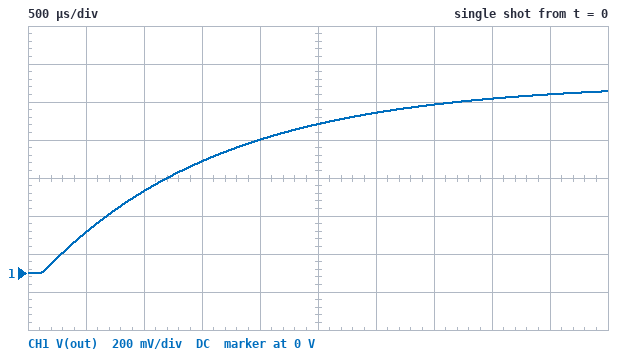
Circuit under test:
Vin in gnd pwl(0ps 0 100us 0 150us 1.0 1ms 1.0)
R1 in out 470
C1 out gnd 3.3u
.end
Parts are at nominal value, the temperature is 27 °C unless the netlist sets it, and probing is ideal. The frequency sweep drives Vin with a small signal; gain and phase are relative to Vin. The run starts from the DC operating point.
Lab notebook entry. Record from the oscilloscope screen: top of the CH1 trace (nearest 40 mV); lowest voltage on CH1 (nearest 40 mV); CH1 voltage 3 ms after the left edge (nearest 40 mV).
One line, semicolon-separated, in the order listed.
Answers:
960 mV; 0 V; 840 mV
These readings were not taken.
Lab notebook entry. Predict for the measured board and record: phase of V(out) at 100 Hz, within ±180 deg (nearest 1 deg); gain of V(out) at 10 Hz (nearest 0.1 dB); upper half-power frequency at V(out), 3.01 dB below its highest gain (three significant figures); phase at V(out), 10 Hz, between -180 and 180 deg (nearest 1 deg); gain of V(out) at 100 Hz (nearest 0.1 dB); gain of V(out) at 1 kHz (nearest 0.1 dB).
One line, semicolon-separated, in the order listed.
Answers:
-44 deg; 0 dB; 103 Hz; -6 deg; -2.9 dB; -19.8 dB
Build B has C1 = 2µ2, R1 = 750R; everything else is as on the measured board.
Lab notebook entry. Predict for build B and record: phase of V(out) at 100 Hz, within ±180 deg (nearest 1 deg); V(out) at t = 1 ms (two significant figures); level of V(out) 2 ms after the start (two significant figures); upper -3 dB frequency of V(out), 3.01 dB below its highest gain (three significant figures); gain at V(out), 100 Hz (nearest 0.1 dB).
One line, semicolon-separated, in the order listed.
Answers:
-46 deg; 410 mV; 680 mV; 96.5 Hz; -3.2 dB
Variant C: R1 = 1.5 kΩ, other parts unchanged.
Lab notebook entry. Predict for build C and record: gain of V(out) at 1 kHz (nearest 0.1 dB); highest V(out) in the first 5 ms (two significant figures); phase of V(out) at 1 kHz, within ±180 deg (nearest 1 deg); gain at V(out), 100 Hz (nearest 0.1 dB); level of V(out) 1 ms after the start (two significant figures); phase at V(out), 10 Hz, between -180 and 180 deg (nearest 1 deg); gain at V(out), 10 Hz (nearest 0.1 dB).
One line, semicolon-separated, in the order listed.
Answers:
-29.9 dB; 630 mV; -88 deg; -10.3 dB; 160 mV; -17 deg; -0.4 dB
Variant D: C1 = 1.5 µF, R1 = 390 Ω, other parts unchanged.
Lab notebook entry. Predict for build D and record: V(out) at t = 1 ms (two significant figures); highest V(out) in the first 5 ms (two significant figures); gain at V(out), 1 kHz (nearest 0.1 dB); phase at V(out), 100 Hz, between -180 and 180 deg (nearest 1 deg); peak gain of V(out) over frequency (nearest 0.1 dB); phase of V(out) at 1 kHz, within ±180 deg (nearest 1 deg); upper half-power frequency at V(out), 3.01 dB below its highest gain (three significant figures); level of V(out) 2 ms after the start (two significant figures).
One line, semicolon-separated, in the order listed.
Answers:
780 mV; 1.0 V; -11.6 dB; -20 deg; 0 dB; -75 deg; 272 Hz; 960 mV
